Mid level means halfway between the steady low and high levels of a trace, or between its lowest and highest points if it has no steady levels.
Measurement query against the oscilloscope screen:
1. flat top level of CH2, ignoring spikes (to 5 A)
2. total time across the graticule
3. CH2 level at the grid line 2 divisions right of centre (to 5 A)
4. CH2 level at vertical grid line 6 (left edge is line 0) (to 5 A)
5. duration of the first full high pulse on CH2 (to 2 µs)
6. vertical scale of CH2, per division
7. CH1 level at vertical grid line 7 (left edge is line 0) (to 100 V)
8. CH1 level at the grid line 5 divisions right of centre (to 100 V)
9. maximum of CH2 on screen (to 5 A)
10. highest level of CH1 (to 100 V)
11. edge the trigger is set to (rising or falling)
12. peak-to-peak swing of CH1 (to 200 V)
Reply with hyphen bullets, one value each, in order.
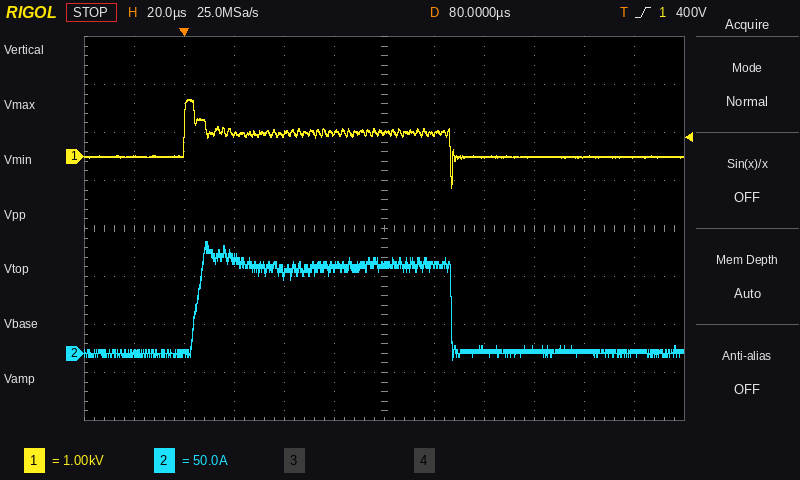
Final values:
- 90 A
- 240 µs
- 5 A
- 90 A
- 102 µs
- 50 A
- 500 V
- 0.0 kV
- 115 A
- 1.2 kV
- rising
- 1.8 kV
